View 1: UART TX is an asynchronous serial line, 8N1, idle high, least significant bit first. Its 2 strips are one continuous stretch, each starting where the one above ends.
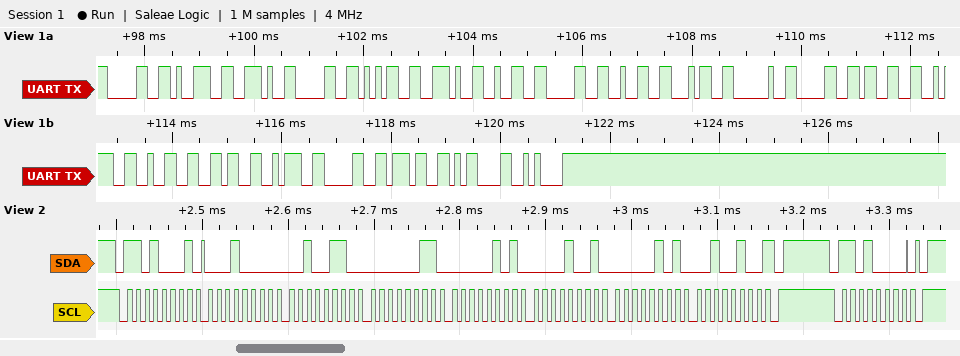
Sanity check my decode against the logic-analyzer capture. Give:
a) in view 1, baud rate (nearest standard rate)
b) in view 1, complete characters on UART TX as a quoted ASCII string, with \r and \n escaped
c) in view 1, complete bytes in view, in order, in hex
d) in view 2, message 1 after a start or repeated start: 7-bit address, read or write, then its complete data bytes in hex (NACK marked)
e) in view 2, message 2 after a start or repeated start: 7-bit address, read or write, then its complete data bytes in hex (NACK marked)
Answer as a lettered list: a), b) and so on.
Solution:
a) 9600 baud
b) "09.05.2024 03:26:07\r\n"
c) 30 39 2E 30 35 2E 32 30 32 34 20 30 33 3A 32 36 3A 30 37 0D 0A
d) 0x68 read: 10 26 03 05 09 05 24 NACK
e) 0x68 write
